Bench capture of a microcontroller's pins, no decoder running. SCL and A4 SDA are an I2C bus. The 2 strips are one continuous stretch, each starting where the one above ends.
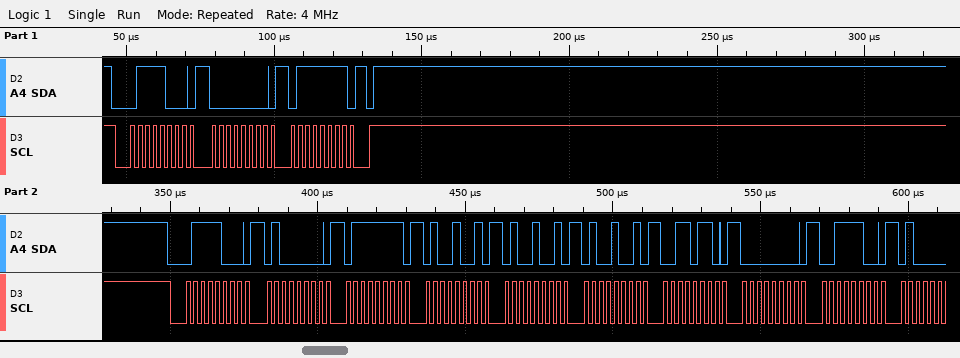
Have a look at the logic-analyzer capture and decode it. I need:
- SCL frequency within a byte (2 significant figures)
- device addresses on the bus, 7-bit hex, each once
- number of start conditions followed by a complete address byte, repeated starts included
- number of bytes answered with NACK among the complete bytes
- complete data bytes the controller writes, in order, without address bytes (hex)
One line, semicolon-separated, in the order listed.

400 kHz; 0x3C; 2; 0; 00 7F 40 7F 49 49 49 36 00 3C
